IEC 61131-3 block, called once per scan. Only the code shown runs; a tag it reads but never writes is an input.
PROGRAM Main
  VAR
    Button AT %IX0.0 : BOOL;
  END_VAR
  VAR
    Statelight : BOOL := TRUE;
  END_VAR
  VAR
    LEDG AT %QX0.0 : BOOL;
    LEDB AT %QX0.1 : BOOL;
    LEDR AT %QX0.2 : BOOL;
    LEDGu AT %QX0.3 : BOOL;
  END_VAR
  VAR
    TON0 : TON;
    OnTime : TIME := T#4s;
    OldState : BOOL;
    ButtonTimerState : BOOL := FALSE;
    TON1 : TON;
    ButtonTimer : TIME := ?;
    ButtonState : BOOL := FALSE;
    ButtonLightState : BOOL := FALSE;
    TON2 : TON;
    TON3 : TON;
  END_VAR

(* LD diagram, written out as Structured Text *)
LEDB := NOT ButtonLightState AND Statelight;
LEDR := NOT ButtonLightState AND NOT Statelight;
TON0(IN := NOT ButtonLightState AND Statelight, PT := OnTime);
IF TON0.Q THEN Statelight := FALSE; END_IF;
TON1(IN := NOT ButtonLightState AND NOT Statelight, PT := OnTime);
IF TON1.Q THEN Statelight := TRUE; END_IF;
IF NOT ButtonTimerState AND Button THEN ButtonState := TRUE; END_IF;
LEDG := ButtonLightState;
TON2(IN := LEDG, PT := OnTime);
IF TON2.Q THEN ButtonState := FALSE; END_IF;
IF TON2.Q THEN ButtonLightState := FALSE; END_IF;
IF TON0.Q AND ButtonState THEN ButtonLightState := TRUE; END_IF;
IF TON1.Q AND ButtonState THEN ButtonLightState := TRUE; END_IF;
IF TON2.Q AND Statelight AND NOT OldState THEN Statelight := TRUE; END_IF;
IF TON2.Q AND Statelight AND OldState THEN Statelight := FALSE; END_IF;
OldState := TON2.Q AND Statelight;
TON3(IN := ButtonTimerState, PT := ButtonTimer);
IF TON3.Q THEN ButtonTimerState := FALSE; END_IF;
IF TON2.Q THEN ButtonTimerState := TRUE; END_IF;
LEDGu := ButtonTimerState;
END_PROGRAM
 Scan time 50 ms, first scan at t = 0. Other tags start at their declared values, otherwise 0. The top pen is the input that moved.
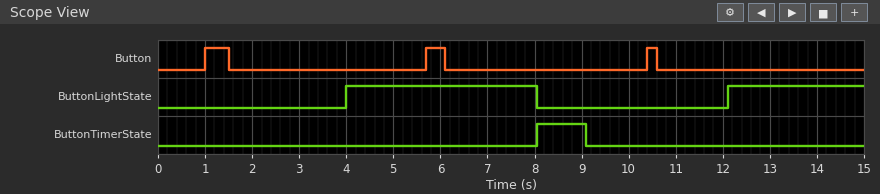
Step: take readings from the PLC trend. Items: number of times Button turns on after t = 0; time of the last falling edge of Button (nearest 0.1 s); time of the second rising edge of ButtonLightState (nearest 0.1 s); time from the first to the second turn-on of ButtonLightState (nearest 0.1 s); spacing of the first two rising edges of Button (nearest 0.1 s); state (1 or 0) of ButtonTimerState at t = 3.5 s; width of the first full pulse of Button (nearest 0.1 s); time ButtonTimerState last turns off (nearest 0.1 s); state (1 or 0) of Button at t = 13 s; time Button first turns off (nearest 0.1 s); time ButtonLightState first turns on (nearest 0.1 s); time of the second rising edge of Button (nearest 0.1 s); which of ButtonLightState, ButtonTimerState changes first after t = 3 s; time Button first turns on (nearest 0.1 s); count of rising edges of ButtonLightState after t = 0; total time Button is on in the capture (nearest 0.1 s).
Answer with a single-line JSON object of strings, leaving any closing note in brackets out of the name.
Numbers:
{"number of times Button turns on after t = 0": "3", "time of the last falling edge of Button": "10.6 s", "time of the second rising edge of ButtonLightState": "12.1 s", "time from the first to the second turn-on of ButtonLightState": "8.1 s", "spacing of the first two rising edges of Button": "4.7 s", "state (1 or 0) of ButtonTimerState at t = 3.5 s": "0", "width of the first full pulse of Button": "0.5 s", "time ButtonTimerState last turns off": "9.1 s", "state (1 or 0) of Button at t = 13 s": "0", "time Button first turns off": "1.5 s", "time ButtonLightState first turns on": "4.0 s", "time of the second rising edge of Button": "5.7 s", "which of ButtonLightState, ButtonTimerState changes first after t = 3 s": "ButtonLightState", "time Button first turns on": "1.0 s", "count of rising edges of ButtonLightState after t = 0": "2", "total time Button is on in the capture": "1.1 s"}
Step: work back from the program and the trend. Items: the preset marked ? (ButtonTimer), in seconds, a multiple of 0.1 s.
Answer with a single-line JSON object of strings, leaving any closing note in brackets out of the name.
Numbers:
{"the preset marked ? (ButtonTimer), in seconds, a multiple of 0.1 s": "1.0 s"}
